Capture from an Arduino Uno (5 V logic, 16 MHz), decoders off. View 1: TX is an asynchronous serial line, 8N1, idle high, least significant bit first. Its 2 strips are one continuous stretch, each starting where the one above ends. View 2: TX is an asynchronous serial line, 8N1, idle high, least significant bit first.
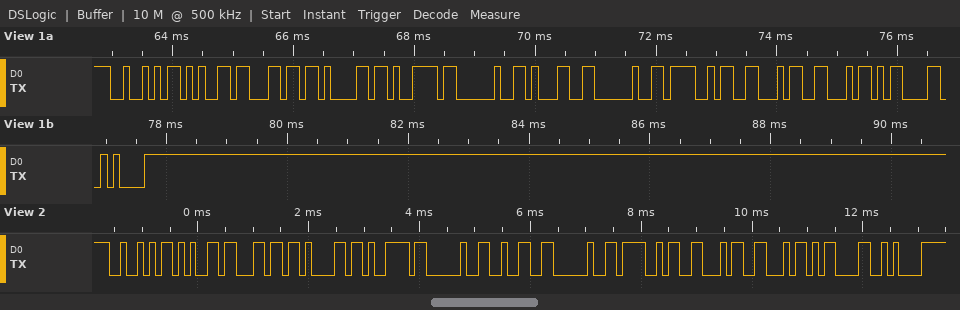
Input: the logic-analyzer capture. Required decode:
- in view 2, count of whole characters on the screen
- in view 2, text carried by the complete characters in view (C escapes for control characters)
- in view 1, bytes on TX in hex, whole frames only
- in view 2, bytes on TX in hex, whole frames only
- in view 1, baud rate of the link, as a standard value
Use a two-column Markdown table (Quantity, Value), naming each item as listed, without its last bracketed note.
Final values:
| Quantity | Value |
|---|---|
| in view 2, count of whole characters on the screen | 13 |
| in view 2, text carried by the complete characters in view | "Relay 2 OFF\r\n" |
| in view 1, bytes on TX in hex, whole frames only | 52 65 6C 61 79 20 31 20 4F 46 46 0D 0A |
| in view 2, bytes on TX in hex, whole frames only | 52 65 6C 61 79 20 32 20 4F 46 46 0D 0A |
| in view 1, baud rate of the link, as a standard value | 9600 baud |
